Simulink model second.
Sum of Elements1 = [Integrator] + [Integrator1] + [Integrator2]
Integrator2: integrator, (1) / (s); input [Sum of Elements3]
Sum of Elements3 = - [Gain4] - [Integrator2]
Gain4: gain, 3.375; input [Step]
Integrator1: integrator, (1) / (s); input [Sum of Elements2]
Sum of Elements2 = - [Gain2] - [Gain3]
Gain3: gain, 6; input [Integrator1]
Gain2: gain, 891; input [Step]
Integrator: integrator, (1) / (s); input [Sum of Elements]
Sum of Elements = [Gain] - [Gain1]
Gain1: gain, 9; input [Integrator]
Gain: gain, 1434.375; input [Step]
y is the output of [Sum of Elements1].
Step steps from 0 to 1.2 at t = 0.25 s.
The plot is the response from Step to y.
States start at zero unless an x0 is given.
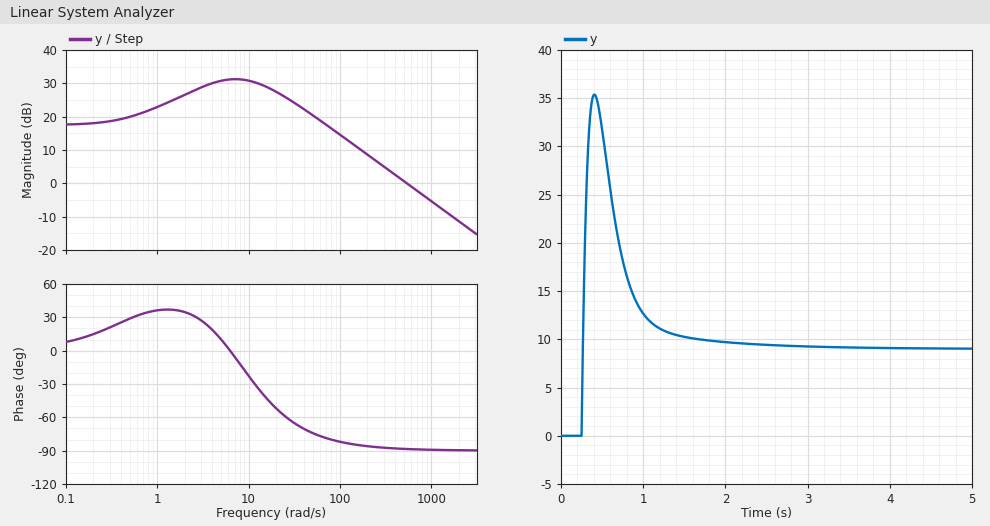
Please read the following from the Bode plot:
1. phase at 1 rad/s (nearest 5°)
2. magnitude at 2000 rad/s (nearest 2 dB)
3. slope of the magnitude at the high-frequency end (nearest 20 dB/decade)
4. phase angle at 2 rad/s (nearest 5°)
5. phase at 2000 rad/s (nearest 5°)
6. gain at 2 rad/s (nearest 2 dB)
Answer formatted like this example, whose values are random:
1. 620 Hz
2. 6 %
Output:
1. 35°
2. -12 dB
3. -20 dB/decade
4. 35°
5. -90°
6. 26 dB
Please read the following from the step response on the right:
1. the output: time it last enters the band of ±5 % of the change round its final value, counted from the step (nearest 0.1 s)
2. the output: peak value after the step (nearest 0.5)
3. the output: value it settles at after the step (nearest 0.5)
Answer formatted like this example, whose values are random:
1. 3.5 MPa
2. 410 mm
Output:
1. 2.2 s
2. 35.5
3. 9.0
